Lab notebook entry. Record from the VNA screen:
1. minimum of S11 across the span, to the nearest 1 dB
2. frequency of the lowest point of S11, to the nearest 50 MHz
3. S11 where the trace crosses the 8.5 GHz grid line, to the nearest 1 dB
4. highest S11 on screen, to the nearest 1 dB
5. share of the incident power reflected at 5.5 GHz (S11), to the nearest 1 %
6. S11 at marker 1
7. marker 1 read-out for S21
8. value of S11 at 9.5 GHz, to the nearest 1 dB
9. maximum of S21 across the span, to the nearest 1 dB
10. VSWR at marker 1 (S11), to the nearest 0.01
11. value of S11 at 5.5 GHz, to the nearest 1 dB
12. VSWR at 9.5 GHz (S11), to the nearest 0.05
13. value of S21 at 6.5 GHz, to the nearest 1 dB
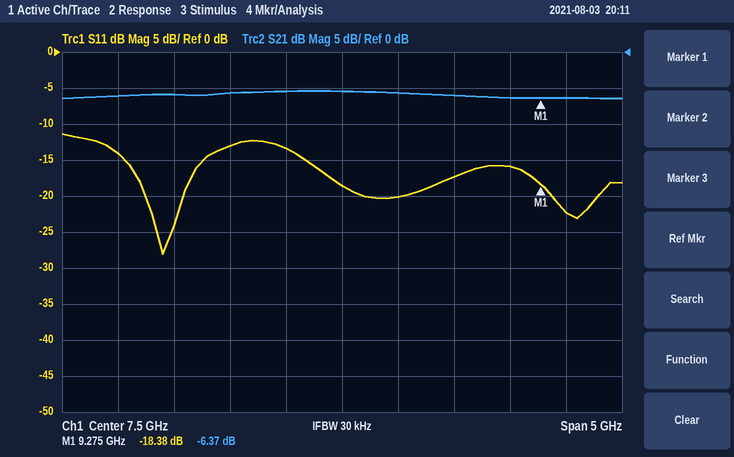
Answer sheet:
-28 dB
5.90 GHz
-17 dB
-11 dB
4 %
-18.38 dB
-6.37 dB
-22 dB
-5 dB
1.27
-14 dB
1.15
-6 dB
